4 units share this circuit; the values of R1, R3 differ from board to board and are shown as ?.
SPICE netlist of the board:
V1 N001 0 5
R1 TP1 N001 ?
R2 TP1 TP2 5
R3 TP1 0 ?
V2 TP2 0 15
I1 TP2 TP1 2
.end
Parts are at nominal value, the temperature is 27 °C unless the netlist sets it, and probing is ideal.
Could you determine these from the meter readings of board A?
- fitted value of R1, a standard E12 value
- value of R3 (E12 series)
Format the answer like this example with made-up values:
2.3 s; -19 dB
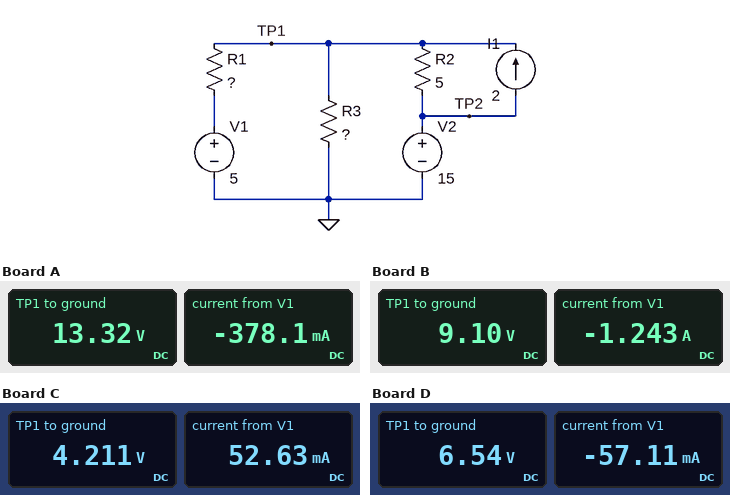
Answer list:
22 Ω; 6.8 Ω
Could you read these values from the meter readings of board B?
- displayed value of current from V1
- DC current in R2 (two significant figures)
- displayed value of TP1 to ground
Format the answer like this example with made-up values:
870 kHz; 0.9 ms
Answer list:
-1.243 A; 1.2 A; 9.10 V
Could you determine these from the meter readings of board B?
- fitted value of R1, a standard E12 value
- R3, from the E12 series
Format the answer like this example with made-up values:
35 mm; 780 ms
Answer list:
3.3 Ω; 4.7 Ω
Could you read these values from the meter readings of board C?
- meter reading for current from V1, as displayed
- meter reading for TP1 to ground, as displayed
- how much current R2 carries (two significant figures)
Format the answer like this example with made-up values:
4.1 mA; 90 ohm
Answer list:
52.63 mA; 4.211 V; 2.2 A
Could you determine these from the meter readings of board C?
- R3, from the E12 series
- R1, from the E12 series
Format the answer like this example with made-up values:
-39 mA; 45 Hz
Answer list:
1 Ω; 15 Ω
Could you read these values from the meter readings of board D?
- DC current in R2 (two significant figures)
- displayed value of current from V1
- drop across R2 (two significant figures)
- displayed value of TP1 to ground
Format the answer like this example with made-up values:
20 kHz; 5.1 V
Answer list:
1.7 A; -57.11 mA; 8.5 V; 6.54 V
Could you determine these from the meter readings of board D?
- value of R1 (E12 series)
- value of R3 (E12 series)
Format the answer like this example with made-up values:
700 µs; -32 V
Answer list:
27 Ω; 1.8 Ω
